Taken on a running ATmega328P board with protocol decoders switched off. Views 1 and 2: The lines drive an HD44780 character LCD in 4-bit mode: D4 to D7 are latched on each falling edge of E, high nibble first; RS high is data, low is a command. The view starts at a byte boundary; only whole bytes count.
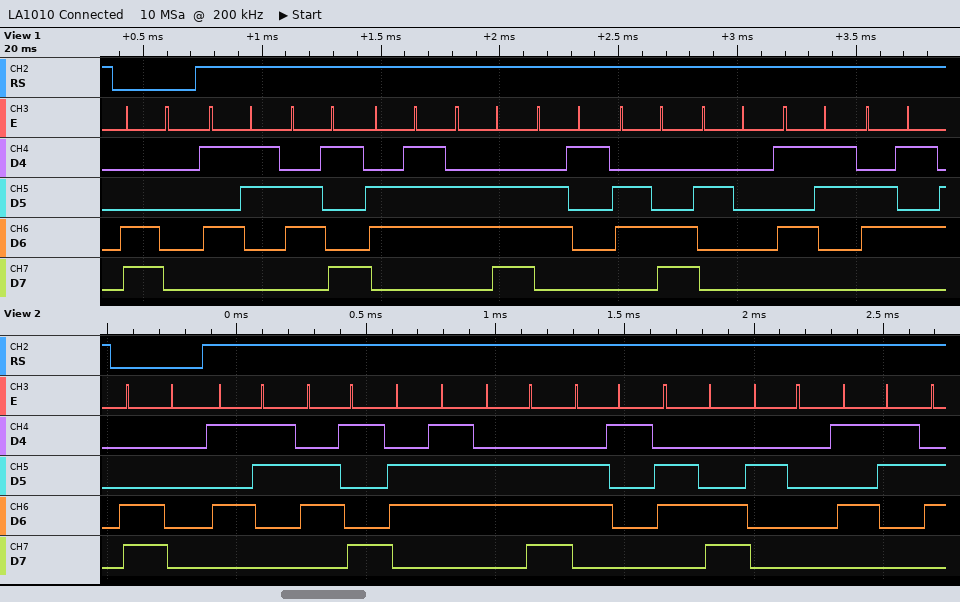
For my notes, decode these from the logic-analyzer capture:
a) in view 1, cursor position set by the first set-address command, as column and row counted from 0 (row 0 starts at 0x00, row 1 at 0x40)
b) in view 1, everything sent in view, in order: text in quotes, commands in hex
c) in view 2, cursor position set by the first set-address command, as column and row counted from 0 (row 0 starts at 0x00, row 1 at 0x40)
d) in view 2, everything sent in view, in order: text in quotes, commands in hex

column 0, row 1
0xC0 "Signal Se"
column 0, row 1
0xC0 "Signal S"
